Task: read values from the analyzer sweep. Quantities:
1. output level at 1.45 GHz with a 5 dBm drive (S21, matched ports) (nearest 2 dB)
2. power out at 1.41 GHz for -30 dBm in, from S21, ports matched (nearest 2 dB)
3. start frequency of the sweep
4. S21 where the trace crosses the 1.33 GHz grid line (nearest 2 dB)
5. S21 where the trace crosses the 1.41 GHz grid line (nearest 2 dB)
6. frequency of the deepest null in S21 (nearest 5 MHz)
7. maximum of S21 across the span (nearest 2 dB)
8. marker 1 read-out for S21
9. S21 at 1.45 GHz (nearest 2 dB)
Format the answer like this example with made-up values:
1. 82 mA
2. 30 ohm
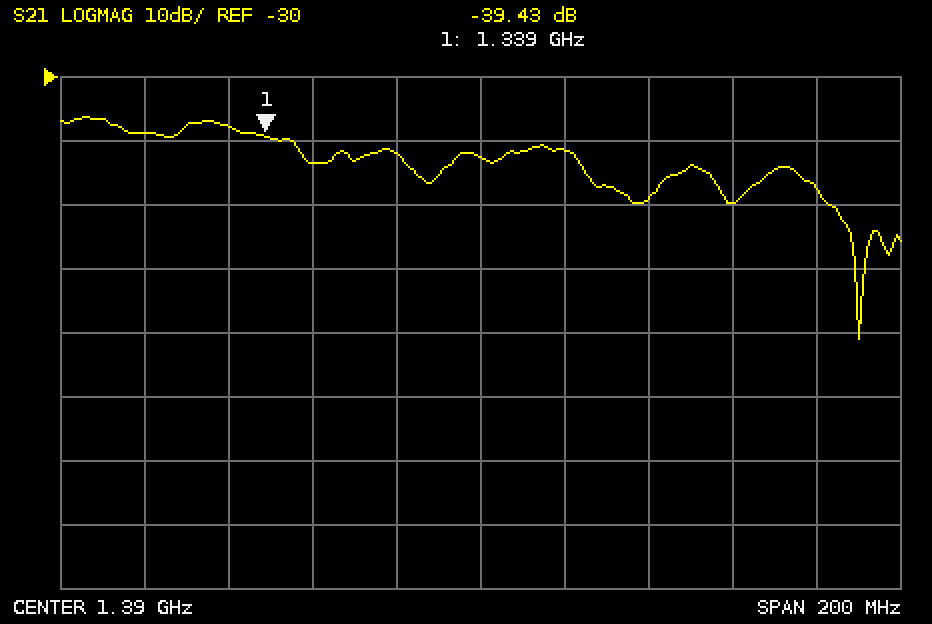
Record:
1. -44 dBm
2. -72 dBm
3. 1.29 GHz
4. -38 dB
5. -42 dB
6. 1.480 GHz
7. -36 dB
8. -39.43 dB
9. -50 dB
